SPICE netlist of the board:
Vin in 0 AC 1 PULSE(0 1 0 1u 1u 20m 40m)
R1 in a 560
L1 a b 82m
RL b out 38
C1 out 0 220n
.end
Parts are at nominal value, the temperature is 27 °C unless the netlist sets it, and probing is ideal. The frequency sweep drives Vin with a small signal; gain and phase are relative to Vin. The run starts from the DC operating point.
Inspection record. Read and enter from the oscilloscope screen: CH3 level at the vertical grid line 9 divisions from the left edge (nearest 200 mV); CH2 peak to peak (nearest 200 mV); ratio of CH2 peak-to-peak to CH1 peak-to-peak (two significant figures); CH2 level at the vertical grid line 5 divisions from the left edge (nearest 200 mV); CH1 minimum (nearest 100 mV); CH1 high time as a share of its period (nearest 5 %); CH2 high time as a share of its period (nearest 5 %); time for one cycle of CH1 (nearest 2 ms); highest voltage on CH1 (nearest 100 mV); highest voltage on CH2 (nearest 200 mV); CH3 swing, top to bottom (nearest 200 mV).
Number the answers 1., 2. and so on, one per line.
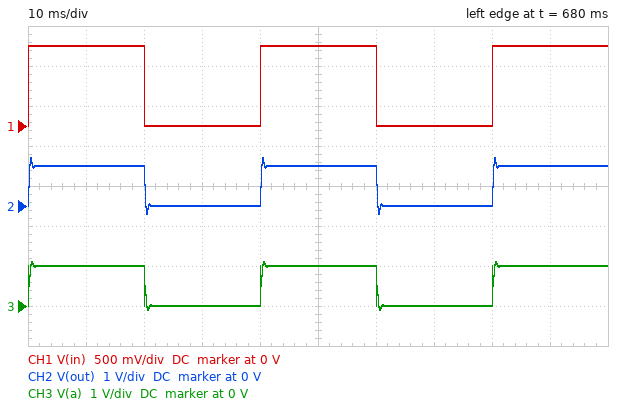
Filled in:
1. 1.0 V
2. 1.4 V
3. 1.4
4. 1.0 V
5. 0 V
6. 50 %
7. 50 %
8. 40 ms
9. 1.0 V
10. 1.2 V
11. 1.2 V
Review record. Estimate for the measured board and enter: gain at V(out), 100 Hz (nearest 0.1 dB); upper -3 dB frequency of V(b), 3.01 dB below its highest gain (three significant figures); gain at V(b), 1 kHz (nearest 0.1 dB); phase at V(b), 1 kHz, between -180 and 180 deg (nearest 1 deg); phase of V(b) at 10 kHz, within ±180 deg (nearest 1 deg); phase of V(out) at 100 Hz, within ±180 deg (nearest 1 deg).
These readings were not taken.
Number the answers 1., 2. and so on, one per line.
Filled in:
1. 0 dB
2. 1.39 kHz
3. 1.2 dB
4. -68 deg
5. -146 deg
6. -5 deg
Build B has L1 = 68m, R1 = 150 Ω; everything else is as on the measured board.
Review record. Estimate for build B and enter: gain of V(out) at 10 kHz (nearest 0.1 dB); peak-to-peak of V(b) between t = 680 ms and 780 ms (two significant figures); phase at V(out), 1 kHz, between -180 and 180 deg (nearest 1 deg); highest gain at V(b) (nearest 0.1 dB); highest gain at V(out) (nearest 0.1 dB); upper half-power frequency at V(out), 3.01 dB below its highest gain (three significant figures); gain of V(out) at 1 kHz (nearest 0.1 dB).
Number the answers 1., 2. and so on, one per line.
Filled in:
1. -35.3 dB
2. 2.2 V
3. -32 deg
4. 9.6 dB
5. 9.5 dB
6. 1.47 kHz
7. 6.3 dB
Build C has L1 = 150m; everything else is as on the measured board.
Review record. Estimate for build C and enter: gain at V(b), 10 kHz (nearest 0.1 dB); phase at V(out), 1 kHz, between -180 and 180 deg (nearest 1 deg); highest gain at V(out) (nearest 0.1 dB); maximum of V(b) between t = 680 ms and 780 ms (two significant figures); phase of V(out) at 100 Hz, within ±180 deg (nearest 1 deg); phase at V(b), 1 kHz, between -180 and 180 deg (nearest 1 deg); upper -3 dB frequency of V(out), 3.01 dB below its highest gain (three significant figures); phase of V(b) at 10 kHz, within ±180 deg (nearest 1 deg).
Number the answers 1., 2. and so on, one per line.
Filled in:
1. -41.2 dB
2. -110 deg
3. 3.4 dB
4. 1.3 V
5. -5 deg
6. -107 deg
7. 1.04 kHz
8. -149 deg
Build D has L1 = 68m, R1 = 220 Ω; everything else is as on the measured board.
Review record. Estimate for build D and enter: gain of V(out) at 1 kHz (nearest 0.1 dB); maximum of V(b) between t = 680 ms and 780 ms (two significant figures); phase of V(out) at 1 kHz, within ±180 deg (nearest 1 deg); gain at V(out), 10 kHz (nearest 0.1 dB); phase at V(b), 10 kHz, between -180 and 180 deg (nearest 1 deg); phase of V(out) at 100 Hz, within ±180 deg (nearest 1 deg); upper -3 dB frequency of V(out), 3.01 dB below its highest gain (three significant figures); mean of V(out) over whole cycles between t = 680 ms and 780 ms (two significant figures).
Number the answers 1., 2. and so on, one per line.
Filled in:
1. 5.3 dB
2. 1.5 V
3. -41 deg
4. -35.3 dB
5. -149 deg
6. -2 deg
7. 1.51 kHz
8. 500 mV
